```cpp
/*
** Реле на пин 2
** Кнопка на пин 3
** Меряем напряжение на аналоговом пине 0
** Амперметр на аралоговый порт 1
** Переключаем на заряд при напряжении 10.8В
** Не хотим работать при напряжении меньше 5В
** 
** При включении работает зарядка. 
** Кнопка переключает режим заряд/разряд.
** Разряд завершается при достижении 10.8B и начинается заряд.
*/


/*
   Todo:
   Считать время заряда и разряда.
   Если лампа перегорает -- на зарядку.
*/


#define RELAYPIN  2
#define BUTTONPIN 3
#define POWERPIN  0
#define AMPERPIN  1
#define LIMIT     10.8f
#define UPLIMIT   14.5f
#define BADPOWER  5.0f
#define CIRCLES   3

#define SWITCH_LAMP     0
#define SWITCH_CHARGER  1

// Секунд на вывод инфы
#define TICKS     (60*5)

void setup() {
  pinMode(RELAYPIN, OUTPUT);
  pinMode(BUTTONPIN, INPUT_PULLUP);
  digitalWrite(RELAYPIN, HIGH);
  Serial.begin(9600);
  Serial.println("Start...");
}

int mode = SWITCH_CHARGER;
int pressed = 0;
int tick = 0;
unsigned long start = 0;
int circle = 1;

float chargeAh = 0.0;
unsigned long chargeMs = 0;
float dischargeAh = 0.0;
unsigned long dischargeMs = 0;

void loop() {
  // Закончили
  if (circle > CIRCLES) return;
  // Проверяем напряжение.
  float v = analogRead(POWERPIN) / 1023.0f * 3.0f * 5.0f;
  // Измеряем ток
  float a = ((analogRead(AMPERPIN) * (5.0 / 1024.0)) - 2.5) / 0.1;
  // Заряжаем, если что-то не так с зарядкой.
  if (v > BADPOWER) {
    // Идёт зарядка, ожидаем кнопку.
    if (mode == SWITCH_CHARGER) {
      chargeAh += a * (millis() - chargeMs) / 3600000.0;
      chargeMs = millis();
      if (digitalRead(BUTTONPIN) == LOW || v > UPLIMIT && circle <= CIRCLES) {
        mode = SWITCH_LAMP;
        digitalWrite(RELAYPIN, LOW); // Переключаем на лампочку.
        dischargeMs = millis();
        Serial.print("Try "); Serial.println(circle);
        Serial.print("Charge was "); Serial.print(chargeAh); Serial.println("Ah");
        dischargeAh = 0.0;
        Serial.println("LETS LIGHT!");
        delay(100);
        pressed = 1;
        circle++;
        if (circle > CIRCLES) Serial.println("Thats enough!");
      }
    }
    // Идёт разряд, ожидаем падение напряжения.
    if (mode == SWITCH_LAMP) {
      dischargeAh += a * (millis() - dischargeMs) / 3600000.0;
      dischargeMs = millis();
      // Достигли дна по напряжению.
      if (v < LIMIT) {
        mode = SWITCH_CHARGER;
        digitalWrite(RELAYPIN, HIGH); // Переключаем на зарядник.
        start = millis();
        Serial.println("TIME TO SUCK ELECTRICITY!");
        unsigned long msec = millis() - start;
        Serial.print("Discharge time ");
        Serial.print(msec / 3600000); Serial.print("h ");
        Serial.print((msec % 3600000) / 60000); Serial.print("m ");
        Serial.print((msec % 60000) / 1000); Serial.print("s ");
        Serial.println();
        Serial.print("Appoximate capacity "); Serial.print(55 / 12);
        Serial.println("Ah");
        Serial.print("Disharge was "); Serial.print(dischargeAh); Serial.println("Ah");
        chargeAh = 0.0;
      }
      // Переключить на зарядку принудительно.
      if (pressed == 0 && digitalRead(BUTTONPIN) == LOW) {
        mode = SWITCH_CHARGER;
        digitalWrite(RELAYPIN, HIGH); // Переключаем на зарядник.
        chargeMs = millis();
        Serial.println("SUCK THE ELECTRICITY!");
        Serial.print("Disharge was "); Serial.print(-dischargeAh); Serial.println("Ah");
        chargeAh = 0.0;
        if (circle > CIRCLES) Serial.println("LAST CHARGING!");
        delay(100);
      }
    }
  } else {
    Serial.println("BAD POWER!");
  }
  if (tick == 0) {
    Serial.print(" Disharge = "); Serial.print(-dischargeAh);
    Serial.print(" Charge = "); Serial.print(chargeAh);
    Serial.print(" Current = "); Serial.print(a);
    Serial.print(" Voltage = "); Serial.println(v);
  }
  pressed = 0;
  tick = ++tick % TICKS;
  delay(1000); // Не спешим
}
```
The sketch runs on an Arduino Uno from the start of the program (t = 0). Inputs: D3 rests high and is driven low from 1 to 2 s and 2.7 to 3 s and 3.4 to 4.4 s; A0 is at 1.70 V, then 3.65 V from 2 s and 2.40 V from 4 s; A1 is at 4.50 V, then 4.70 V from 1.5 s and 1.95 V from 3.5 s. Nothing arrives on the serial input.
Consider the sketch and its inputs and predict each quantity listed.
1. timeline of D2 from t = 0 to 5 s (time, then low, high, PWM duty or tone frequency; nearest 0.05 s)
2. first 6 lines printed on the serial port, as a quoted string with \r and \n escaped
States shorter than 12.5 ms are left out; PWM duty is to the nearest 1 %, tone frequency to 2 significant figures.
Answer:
0 s high; 1 s low; 1.1 s high; 4.15 s low; 4.25 s high
"Start...\r\n Disharge = 0.00 Charge = 0.00 Current = 19.97 Voltage = 5.10\r\nTry 1\r\nCharge was 0.01Ah\r\nLETS LIGHT!\r\nTIME TO SUCK ELECTRICITY!\r\n"
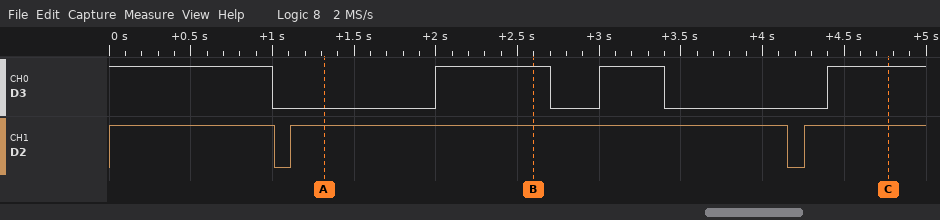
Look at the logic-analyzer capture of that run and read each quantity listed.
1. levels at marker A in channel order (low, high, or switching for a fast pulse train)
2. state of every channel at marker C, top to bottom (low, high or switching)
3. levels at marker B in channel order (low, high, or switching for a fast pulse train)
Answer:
D3 low, D2 high
D3 high, D2 high
D3 high, D2 high
